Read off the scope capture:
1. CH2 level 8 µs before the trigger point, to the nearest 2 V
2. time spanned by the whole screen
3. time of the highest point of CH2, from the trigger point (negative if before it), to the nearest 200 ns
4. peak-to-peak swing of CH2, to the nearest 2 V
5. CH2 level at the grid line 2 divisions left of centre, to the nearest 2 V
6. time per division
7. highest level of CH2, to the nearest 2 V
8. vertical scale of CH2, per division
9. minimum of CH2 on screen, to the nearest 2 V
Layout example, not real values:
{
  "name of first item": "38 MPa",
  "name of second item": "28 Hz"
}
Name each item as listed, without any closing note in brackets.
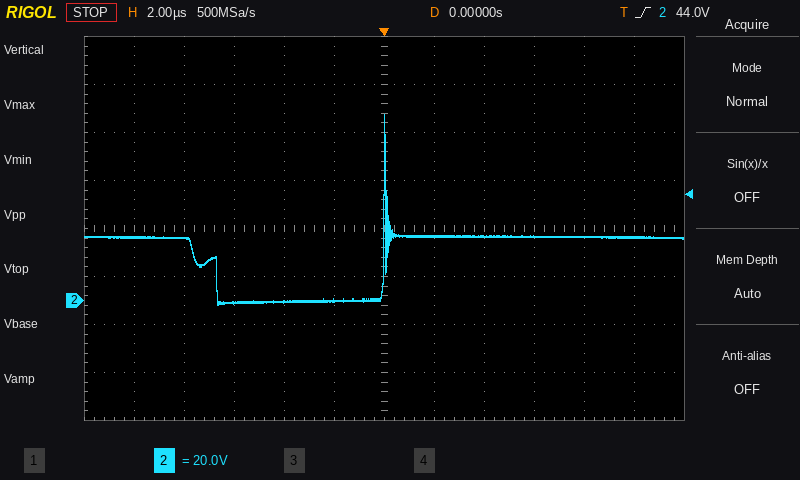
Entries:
{
  "CH2 level 8 µs before the trigger point, to the nearest 2 V": "26 V",
  "time spanned by the whole screen": "24 µs",
  "time of the highest point of CH2, from the trigger point (negative if before it), to the nearest 200 ns": "0.0 µs",
  "peak-to-peak swing of CH2, to the nearest 2 V": "80 V",
  "CH2 level at the grid line 2 divisions left of centre, to the nearest 2 V": "0 V",
  "time per division": "2 µs",
  "highest level of CH2, to the nearest 2 V": "78 V",
  "vertical scale of CH2, per division": "20 V",
  "minimum of CH2 on screen, to the nearest 2 V": "-2 V"
}
